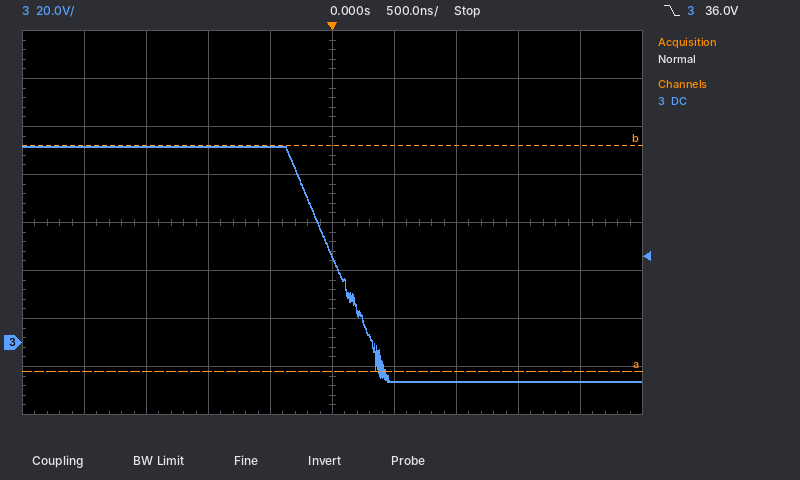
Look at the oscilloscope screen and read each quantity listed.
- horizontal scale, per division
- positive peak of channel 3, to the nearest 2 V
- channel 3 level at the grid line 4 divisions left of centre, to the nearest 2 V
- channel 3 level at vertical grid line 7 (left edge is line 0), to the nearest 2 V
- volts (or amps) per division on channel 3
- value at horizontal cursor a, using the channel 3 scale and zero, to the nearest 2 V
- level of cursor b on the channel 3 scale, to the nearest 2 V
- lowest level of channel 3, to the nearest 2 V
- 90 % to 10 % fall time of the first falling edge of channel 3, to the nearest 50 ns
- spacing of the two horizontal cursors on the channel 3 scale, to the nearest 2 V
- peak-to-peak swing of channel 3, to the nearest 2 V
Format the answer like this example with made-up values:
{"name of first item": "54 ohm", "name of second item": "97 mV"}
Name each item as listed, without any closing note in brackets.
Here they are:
{"horizontal scale, per division": "500 ns", "positive peak of channel 3, to the nearest 2 V": "82 V", "channel 3 level at the grid line 4 divisions left of centre, to the nearest 2 V": "82 V", "channel 3 level at vertical grid line 7 (left edge is line 0), to the nearest 2 V": "-16 V", "volts (or amps) per division on channel 3": "20 V", "value at horizontal cursor a, using the channel 3 scale and zero, to the nearest 2 V": "-12 V", "level of cursor b on the channel 3 scale, to the nearest 2 V": "82 V", "lowest level of channel 3, to the nearest 2 V": "-16 V", "90 % to 10 % fall time of the first falling edge of channel 3, to the nearest 50 ns": "650 ns", "spacing of the two horizontal cursors on the channel 3 scale, to the nearest 2 V": "94 V", "peak-to-peak swing of channel 3, to the nearest 2 V": "98 V"}
